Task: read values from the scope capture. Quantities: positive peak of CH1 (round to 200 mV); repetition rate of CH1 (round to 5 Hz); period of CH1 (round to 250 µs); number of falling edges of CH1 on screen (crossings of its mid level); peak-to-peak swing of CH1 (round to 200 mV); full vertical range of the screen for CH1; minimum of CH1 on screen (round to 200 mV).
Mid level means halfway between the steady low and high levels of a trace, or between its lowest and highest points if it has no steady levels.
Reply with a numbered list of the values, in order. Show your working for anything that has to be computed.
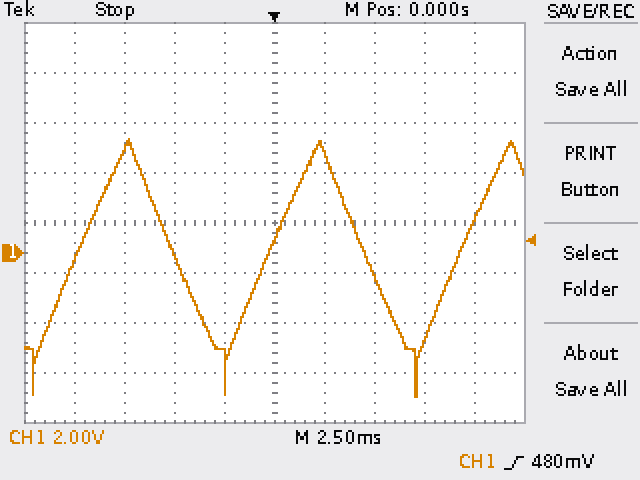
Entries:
1. 4.6 V
2. 1 / 9.50 ms ≈ 105 Hz
3. 9.50 ms
4. 2
5. 4.6 V − (-5.8 V) = 10.4 V
6. 16 V
7. -5.8 V
